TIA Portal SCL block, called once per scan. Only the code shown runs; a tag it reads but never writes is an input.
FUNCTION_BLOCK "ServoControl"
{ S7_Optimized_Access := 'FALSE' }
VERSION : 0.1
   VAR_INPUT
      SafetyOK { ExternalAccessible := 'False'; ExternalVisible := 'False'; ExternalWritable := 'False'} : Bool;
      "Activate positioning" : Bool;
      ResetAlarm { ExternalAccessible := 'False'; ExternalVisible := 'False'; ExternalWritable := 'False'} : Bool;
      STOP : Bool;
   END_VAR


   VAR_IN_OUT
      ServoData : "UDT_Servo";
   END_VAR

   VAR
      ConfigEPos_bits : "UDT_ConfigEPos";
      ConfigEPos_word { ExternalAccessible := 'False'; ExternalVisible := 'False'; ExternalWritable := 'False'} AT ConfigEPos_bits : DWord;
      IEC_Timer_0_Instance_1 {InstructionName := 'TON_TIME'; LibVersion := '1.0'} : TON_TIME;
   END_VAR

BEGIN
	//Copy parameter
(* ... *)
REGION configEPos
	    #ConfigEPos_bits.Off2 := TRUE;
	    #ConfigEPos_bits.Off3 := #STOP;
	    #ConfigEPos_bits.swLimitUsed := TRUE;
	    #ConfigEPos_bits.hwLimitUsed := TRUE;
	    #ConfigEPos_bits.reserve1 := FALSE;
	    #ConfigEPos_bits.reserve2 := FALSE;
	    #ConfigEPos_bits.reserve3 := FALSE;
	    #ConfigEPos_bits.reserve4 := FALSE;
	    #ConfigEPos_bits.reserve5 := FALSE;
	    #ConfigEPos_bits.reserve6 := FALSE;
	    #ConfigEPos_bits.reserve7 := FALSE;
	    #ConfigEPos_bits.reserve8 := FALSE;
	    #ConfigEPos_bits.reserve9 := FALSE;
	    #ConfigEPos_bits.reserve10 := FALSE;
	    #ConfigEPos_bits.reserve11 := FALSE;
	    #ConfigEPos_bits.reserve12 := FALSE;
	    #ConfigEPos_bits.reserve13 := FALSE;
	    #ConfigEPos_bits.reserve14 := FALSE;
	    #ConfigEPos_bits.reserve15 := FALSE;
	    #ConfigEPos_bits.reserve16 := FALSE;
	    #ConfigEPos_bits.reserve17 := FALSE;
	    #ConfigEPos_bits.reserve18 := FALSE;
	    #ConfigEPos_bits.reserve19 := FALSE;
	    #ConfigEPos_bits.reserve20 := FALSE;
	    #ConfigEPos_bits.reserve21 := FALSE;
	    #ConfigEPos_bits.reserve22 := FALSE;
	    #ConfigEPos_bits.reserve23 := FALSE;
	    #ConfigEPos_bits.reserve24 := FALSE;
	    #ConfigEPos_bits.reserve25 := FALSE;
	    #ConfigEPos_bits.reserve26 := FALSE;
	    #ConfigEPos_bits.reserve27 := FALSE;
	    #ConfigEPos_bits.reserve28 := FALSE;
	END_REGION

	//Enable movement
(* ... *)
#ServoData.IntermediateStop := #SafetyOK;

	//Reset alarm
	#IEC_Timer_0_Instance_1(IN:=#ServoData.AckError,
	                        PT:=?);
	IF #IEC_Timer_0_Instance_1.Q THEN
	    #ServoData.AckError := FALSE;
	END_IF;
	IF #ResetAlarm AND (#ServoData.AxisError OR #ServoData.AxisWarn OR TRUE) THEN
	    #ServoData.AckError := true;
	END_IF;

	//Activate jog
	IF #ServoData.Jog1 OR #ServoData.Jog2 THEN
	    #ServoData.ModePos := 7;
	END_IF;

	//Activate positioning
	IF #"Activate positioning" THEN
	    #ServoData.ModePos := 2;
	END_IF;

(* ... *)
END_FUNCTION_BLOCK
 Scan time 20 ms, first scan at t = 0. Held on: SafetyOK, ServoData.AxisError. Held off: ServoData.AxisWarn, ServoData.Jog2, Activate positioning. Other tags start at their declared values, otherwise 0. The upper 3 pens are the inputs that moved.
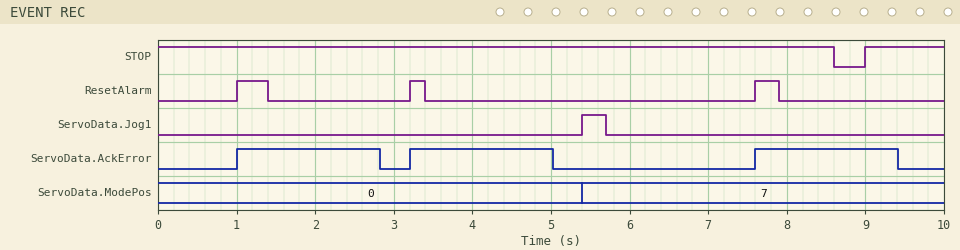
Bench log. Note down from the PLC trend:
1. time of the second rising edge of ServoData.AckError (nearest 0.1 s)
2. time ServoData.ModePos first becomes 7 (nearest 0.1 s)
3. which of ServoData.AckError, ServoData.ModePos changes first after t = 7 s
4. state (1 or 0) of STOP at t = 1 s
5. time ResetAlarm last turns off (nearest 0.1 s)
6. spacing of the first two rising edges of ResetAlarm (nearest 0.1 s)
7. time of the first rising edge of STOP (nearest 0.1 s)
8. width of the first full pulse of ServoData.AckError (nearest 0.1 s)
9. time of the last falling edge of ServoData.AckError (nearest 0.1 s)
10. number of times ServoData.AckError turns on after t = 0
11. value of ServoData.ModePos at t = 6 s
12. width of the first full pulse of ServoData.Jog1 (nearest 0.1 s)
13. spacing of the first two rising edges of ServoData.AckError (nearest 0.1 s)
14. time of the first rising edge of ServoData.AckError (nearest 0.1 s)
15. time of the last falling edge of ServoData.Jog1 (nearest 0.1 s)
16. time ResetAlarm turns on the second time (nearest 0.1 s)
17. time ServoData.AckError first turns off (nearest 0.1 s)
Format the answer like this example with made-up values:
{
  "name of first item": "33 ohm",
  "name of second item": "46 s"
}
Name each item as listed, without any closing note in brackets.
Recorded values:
{
  "time of the second rising edge of ServoData.AckError": "3.2 s",
  "time ServoData.ModePos first becomes 7": "5.4 s",
  "which of ServoData.AckError, ServoData.ModePos changes first after t = 7 s": "ServoData.AckError",
  "state (1 or 0) of STOP at t = 1 s": "1",
  "time ResetAlarm last turns off": "7.9 s",
  "spacing of the first two rising edges of ResetAlarm": "2.2 s",
  "time of the first rising edge of STOP": "9.0 s",
  "width of the first full pulse of ServoData.AckError": "1.8 s",
  "time of the last falling edge of ServoData.AckError": "9.4 s",
  "number of times ServoData.AckError turns on after t = 0": "3",
  "value of ServoData.ModePos at t = 6 s": "7",
  "width of the first full pulse of ServoData.Jog1": "0.3 s",
  "spacing of the first two rising edges of ServoData.AckError": "2.2 s",
  "time of the first rising edge of ServoData.AckError": "1.0 s",
  "time of the last falling edge of ServoData.Jog1": "5.7 s",
  "time ResetAlarm turns on the second time": "3.2 s",
  "time ServoData.AckError first turns off": "2.8 s"
}
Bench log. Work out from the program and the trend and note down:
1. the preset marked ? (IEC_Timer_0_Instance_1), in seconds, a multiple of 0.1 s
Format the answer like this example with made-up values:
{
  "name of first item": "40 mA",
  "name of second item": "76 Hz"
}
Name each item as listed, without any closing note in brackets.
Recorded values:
{
  "the preset marked ? (IEC_Timer_0_Instance_1), in seconds, a multiple of 0.1 s": "1.8 s"
}
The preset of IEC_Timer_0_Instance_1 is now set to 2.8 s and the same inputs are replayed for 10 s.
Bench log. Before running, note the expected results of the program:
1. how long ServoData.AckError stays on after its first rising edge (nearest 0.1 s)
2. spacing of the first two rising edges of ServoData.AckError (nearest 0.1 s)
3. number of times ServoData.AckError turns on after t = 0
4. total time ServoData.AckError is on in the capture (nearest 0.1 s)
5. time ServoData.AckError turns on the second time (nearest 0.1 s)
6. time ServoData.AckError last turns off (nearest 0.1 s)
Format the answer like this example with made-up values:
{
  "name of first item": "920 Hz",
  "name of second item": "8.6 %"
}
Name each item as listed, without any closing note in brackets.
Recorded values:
{
  "how long ServoData.AckError stays on after its first rising edge": "2.8 s",
  "spacing of the first two rising edges of ServoData.AckError": "6.6 s",
  "number of times ServoData.AckError turns on after t = 0": "2",
  "total time ServoData.AckError is on in the capture": "5.2 s",
  "time ServoData.AckError turns on the second time": "7.6 s",
  "time ServoData.AckError last turns off": "3.8 s"
}
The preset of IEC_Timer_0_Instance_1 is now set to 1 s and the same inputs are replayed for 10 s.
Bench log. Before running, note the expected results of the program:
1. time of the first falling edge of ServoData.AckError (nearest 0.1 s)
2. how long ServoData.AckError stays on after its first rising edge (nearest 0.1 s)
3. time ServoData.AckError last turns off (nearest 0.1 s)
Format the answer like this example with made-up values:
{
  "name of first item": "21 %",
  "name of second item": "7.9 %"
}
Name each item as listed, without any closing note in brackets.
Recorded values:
{
  "time of the first falling edge of ServoData.AckError": "2.0 s",
  "how long ServoData.AckError stays on after its first rising edge": "1.0 s",
  "time ServoData.AckError last turns off": "8.6 s"
}
